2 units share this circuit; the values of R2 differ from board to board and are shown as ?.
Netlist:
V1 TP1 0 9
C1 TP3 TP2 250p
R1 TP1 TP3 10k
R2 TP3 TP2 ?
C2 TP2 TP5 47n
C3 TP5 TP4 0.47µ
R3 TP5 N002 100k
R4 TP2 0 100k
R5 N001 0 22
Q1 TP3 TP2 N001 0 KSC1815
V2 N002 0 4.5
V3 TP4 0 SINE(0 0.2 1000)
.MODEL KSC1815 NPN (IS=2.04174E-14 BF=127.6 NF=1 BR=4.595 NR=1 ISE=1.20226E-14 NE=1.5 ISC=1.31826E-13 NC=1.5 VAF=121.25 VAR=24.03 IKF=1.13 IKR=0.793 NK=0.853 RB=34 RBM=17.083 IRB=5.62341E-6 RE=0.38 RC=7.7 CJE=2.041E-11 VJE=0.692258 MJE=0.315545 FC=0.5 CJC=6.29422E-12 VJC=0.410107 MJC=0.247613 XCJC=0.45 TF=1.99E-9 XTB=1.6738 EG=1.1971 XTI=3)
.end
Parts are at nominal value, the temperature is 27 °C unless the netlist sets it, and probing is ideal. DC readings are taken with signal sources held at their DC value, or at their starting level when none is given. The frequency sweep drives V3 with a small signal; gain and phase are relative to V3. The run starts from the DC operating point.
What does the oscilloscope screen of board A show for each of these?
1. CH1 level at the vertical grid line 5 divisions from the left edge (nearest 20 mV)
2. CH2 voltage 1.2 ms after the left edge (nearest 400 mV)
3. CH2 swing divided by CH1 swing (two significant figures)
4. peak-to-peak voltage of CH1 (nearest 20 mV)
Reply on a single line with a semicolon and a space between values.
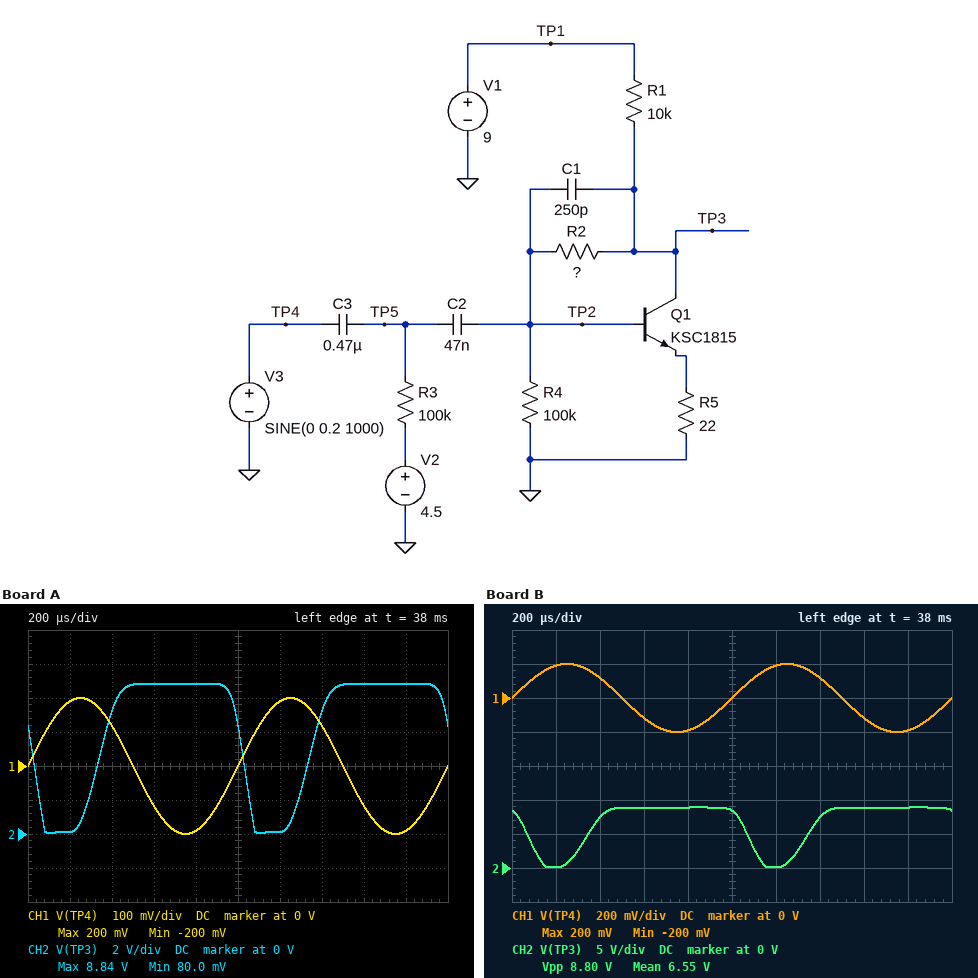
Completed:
0 V; 0 V; 22; 400 mV
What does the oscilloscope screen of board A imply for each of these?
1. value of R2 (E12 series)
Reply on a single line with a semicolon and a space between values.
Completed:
560 kΩ
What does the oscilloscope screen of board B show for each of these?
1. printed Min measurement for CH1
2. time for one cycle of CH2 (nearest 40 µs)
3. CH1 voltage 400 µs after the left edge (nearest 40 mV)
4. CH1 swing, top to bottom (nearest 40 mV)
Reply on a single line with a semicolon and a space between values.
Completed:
-200 mV; 1.00 ms; 120 mV; 400 mV
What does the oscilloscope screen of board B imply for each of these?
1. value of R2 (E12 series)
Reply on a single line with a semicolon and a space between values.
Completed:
820 kΩ
